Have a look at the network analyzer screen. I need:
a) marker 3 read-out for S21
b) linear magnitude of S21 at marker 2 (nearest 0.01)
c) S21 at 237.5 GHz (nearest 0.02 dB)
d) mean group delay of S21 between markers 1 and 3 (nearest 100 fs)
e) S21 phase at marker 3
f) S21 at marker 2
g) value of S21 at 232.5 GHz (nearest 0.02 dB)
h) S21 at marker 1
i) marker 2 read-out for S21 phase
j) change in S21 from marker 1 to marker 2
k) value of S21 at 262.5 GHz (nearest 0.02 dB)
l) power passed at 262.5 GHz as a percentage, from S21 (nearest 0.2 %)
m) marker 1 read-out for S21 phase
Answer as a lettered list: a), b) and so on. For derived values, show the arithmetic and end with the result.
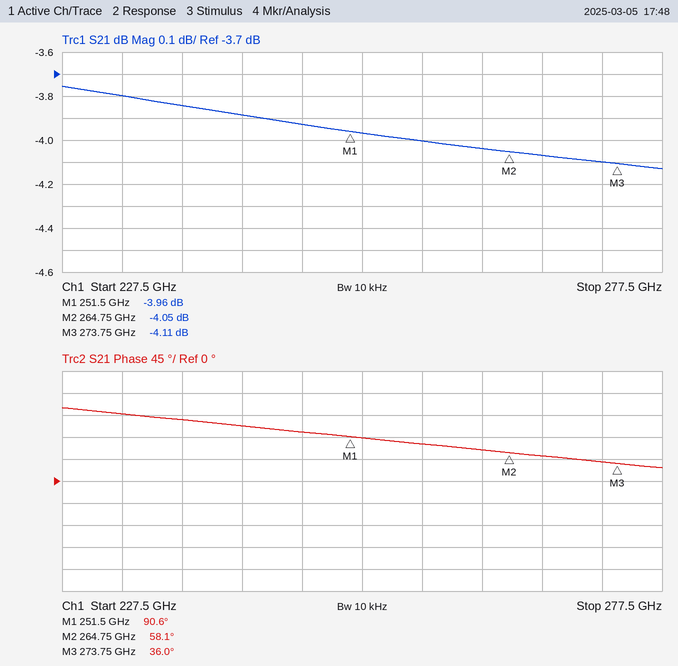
a) -4.11 dB
b) 10^(-4.05/20) ≈ 0.63
c) -3.84 dB
d) −(36° − (90.6°))/(360° × 22.25 GHz) ≈ 6.8 ps
e) 36.0°
f) -4.05 dB
g) -3.80 dB
h) -3.96 dB
i) 58.1°
j) -4.05 − (-3.96) = -0.09 dB
k) -4.04 dB
l) 10^(-4.04/10) ≈ 39.4 %
m) 90.6°
